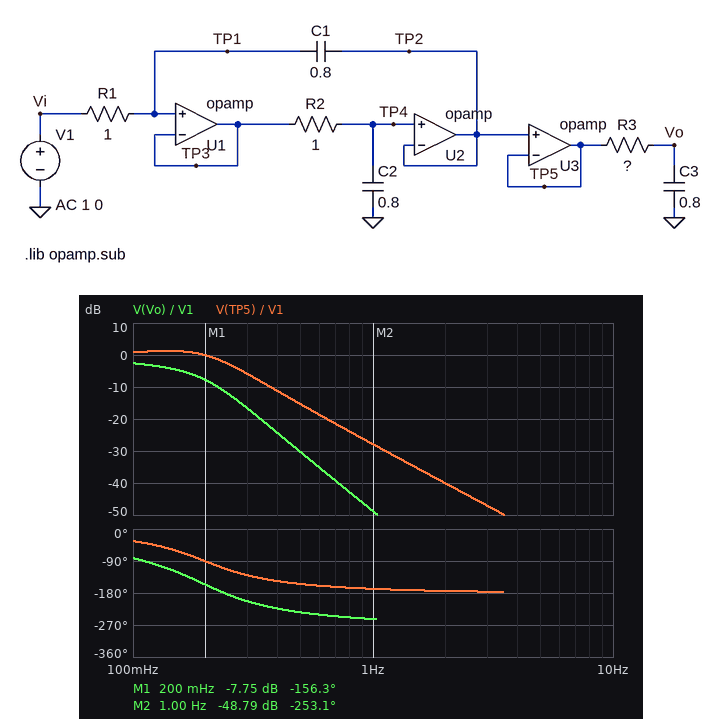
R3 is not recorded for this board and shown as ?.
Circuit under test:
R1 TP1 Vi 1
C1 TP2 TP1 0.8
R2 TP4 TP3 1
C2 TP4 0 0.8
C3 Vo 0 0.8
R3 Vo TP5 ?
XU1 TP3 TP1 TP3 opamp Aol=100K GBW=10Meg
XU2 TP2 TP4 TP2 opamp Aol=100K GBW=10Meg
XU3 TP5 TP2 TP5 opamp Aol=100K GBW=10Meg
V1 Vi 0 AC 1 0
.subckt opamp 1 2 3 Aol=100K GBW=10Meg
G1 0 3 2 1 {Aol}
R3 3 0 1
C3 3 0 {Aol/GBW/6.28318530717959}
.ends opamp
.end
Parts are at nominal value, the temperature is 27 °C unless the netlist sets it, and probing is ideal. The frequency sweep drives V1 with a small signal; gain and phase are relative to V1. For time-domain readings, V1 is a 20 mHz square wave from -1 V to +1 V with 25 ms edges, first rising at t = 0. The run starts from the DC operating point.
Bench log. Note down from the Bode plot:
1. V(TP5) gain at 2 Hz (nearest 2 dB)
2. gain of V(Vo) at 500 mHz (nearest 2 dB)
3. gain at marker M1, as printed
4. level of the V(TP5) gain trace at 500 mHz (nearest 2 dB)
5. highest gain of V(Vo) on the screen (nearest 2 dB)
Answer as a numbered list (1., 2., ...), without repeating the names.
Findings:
1. -40 dB
2. -30 dB
3. -7.75 dB
4. -16 dB
5. -2 dB
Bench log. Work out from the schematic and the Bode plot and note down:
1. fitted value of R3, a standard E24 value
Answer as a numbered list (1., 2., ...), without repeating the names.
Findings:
1. 2.2 Ω
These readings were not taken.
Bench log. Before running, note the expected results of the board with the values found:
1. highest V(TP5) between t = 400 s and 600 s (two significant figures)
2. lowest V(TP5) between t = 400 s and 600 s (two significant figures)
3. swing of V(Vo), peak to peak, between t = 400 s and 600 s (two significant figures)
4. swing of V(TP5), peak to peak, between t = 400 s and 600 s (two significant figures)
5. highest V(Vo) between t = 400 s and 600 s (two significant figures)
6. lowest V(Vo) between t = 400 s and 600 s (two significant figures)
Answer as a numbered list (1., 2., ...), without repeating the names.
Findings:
1. 1.3 V
2. -1.3 V
3. 2.0 V
4. 2.7 V
5. 1.0 V
6. -1.0 V
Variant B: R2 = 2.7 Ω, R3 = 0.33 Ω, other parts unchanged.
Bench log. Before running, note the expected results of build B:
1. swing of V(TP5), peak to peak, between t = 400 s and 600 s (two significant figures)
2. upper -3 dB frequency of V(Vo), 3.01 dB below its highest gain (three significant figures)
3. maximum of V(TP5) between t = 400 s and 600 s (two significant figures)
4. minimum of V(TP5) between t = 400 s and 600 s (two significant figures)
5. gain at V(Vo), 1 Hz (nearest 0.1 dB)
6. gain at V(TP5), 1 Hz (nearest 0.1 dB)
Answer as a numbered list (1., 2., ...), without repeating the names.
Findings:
1. 2.0 V
2. 100 mHz
3. 1.0 V
4. -1.0 V
5. -42.5 dB
6. -36.7 dB
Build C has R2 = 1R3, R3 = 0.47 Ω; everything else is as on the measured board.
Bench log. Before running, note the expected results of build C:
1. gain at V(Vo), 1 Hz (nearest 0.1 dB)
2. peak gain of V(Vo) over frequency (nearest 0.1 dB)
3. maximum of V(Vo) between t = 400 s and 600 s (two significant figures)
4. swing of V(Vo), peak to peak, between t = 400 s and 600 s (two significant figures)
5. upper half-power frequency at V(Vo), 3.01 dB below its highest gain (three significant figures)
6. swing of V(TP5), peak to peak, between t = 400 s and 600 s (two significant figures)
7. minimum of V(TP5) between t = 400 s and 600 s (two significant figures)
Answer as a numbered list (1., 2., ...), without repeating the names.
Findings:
1. -38.4 dB
2. 0.3 dB
3. 1.2 V
4. 2.4 V
5. 188 mHz
6. 2.5 V
7. -1.2 V
